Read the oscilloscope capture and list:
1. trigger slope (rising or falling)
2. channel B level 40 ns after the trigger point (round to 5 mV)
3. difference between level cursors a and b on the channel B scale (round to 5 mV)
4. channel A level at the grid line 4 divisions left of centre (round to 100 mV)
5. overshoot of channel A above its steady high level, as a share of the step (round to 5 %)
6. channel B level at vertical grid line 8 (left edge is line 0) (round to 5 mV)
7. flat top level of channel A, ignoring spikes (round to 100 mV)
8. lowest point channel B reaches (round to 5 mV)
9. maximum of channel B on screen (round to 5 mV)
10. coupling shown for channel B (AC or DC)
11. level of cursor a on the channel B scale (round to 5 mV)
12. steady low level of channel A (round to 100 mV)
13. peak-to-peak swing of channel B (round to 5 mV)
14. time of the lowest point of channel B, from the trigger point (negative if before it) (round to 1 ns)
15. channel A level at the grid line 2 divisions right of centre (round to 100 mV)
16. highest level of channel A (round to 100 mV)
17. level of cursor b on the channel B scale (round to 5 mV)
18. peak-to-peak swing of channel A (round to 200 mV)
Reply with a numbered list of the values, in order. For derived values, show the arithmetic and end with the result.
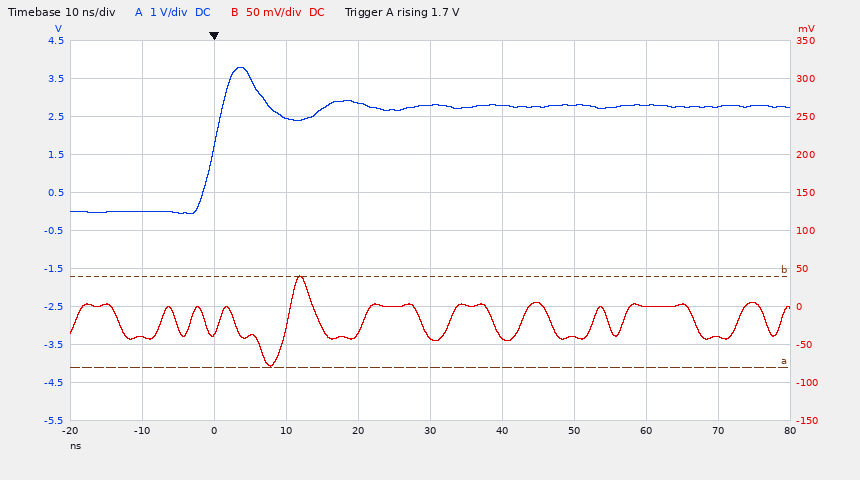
1. rising
2. -40 mV
3. 120 mV
4. 0.0 V
5. 35 %
6. 0 mV
7. 2.8 V
8. -80 mV
9. 40 mV
10. DC
11. -80 mV
12. 0.0 V
13. 40 mV − (-80 mV) = 120 mV
14. +8 ns
15. 2.8 V
16. 3.8 V
17. 40 mV
18. 3.8 V
